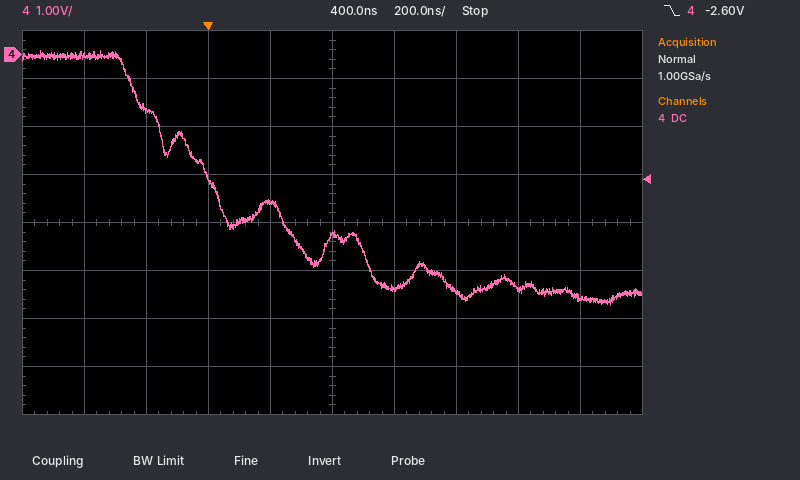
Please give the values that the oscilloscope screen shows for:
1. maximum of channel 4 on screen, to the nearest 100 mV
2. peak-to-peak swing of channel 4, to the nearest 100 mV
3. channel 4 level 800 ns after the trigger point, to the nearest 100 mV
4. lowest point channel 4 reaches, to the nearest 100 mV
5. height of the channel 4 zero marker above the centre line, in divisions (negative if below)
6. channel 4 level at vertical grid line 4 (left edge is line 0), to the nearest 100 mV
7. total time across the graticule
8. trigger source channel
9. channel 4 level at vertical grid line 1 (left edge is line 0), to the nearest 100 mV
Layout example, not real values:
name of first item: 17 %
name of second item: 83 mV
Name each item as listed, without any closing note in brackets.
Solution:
maximum of channel 4 on screen, to the nearest 100 mV: 100 mV
peak-to-peak swing of channel 4, to the nearest 100 mV: 5.3 V
channel 4 level 800 ns after the trigger point, to the nearest 100 mV: -4.9 V
lowest point channel 4 reaches, to the nearest 100 mV: -5.2 V
height of the channel 4 zero marker above the centre line, in divisions: +3.5 div
channel 4 level at vertical grid line 4 (left edge is line 0), to the nearest 100 mV: -3.1 V
total time across the graticule: 2 µs
trigger source channel: channel 4
channel 4 level at vertical grid line 1 (left edge is line 0), to the nearest 100 mV: 0.0 V
